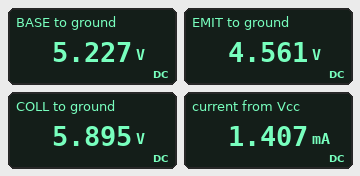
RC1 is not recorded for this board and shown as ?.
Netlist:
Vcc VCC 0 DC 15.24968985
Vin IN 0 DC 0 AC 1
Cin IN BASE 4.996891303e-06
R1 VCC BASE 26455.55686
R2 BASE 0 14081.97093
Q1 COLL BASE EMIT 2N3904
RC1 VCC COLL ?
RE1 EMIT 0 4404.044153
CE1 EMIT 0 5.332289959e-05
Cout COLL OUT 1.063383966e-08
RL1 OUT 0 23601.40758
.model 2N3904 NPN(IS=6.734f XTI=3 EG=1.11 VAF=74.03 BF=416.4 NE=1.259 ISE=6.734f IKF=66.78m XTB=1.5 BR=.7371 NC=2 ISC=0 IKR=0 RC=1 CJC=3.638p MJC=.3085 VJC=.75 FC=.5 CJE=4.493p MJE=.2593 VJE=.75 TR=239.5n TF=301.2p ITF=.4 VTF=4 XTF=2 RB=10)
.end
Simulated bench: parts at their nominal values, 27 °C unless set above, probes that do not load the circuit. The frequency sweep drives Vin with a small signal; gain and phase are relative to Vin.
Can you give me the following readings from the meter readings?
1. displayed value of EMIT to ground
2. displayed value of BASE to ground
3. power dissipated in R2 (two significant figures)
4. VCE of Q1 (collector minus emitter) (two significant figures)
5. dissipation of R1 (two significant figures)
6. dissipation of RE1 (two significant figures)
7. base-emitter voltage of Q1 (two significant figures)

4.561 V
5.227 V
1.9 mW
1.3 V
3.8 mW
4.7 mW
670 mV
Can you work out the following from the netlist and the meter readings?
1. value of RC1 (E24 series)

9.1 kΩ
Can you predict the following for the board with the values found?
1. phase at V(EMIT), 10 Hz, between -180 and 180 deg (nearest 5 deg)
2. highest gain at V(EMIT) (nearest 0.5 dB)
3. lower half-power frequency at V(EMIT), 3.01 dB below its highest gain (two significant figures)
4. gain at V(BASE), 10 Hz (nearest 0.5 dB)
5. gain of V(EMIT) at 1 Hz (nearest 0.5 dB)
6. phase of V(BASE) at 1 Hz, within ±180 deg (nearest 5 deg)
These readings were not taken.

15 deg
-1.0 dB
3.1 Hz
-1.0 dB
-11.5 dB
75 deg
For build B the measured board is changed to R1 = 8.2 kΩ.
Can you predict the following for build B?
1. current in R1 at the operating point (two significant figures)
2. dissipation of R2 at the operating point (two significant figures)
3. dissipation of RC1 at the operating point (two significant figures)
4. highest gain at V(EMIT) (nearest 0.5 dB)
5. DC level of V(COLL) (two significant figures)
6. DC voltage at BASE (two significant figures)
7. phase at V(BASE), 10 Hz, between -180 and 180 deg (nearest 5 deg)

990 µA
3.6 mW
8.5 mW
-21.5 dB
6.5 V
7.1 V
15 deg
